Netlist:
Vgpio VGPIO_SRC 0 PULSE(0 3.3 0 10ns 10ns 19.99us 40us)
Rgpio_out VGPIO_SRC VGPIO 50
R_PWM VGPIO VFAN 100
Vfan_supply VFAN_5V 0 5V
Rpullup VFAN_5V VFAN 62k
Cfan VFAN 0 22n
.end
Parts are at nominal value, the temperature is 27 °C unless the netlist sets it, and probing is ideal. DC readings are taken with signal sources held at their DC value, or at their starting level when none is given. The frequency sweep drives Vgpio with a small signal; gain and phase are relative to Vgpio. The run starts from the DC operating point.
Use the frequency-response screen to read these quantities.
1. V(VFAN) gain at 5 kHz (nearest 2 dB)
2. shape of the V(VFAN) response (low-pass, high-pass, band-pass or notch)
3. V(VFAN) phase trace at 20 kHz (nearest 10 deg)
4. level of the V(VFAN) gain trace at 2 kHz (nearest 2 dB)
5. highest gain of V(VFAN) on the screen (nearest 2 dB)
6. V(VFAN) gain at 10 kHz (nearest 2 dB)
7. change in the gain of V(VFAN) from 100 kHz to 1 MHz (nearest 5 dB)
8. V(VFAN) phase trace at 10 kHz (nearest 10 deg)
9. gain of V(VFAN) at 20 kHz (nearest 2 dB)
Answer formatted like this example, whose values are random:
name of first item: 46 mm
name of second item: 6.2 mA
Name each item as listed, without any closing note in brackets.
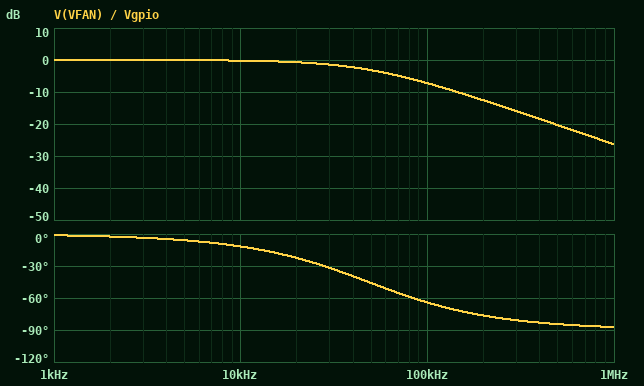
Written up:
V(VFAN) gain at 5 kHz: 0 dB
shape of the V(VFAN) response: low-pass
V(VFAN) phase trace at 20 kHz: -20 deg
level of the V(VFAN) gain trace at 2 kHz: 0 dB
highest gain of V(VFAN) on the screen: 0 dB
V(VFAN) gain at 10 kHz: 0 dB
change in the gain of V(VFAN) from 100 kHz to 1 MHz: -20 dB
V(VFAN) phase trace at 10 kHz: -10 deg
gain of V(VFAN) at 20 kHz: 0 dB
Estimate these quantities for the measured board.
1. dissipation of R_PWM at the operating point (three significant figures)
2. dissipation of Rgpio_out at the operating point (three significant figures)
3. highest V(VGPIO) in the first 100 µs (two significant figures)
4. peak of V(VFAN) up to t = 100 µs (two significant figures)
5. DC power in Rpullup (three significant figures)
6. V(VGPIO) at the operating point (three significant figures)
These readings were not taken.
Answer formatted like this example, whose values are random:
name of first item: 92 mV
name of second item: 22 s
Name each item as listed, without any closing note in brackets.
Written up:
dissipation of R_PWM at the operating point: 647 nW
dissipation of Rgpio_out at the operating point: 324 nW
highest V(VGPIO) in the first 100 µs: 3.3 V
peak of V(VFAN) up to t = 100 µs: 3.3 V
DC power in Rpullup: 401 µW
V(VGPIO) at the operating point: 4.02 mV
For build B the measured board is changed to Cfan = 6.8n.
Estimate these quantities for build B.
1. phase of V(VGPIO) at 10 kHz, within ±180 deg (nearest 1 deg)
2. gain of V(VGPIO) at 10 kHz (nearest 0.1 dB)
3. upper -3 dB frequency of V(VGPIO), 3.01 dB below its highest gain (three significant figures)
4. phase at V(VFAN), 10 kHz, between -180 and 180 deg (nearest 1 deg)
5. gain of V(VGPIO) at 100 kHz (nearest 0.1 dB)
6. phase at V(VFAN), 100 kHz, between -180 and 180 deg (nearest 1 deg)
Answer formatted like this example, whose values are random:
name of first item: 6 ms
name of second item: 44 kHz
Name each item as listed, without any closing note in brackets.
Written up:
phase of V(VGPIO) at 10 kHz, within ±180 deg: -1 deg
gain of V(VGPIO) at 10 kHz: 0 dB
upper -3 dB frequency of V(VGPIO), 3.01 dB below its highest gain: 472 kHz
phase at V(VFAN), 10 kHz, between -180 and 180 deg: -4 deg
gain of V(VGPIO) at 100 kHz: -0.8 dB
phase at V(VFAN), 100 kHz, between -180 and 180 deg: -33 deg
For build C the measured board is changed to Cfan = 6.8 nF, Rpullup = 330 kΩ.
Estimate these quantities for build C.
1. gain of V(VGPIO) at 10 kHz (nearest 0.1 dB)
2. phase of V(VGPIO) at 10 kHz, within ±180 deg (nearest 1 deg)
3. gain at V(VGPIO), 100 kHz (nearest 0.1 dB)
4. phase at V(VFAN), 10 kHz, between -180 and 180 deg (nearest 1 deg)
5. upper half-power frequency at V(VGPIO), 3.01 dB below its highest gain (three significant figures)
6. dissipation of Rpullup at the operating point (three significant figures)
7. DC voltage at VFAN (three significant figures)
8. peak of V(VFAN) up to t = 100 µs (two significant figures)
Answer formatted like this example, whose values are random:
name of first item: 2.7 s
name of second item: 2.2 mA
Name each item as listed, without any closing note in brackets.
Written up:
gain of V(VGPIO) at 10 kHz: 0 dB
phase of V(VGPIO) at 10 kHz, within ±180 deg: -1 deg
gain at V(VGPIO), 100 kHz: -0.8 dB
phase at V(VFAN), 10 kHz, between -180 and 180 deg: -4 deg
upper half-power frequency at V(VGPIO), 3.01 dB below its highest gain: 469 kHz
dissipation of Rpullup at the operating point: 75.7 µW
DC voltage at VFAN: 2.27 mV
peak of V(VFAN) up to t = 100 µs: 3.3 V
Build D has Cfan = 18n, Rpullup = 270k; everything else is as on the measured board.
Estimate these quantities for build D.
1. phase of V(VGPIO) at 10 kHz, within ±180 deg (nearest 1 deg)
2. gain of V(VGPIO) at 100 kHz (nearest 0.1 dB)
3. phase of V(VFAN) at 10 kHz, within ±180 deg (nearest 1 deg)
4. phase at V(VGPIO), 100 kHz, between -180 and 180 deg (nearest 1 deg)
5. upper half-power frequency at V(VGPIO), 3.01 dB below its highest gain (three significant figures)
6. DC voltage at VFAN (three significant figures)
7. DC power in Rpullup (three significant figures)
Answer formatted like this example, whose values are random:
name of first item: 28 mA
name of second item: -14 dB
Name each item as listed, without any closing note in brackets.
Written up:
phase of V(VGPIO) at 10 kHz, within ±180 deg: -3 deg
gain of V(VGPIO) at 100 kHz: -2.3 dB
phase of V(VFAN) at 10 kHz, within ±180 deg: -10 deg
phase at V(VGPIO), 100 kHz, between -180 and 180 deg: -11 deg
upper half-power frequency at V(VGPIO), 3.01 dB below its highest gain: 177 kHz
DC voltage at VFAN: 2.78 mV
DC power in Rpullup: 92.5 µW
